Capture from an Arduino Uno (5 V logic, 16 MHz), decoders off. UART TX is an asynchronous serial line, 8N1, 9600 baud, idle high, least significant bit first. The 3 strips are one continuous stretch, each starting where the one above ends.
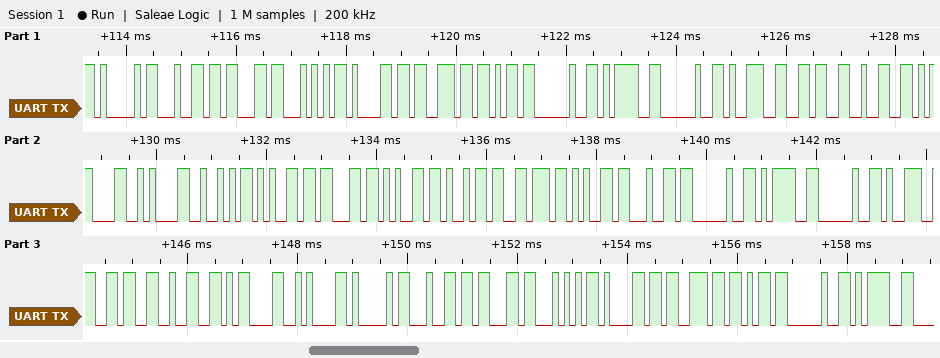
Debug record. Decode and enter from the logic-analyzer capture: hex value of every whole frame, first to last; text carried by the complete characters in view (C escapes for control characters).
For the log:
0x41 0x64 0x63 0x54 0x61 0x73 0x6B 0x20 0x3D 0x20 0x39 0x36 0x32 0x0D 0x0A 0x52 0x65 0x63 0x65 0x69 0x76 0x65 0x64 0x20 0x3D 0x20 0x39 0x36 0x32 0x0D 0x0A 0x41 0x64 0x63 0x54 0x61 0x73 0x6B 0x20 0x3D
"AdcTask = 962\r\nReceived = 962\r\nAdcTask ="
